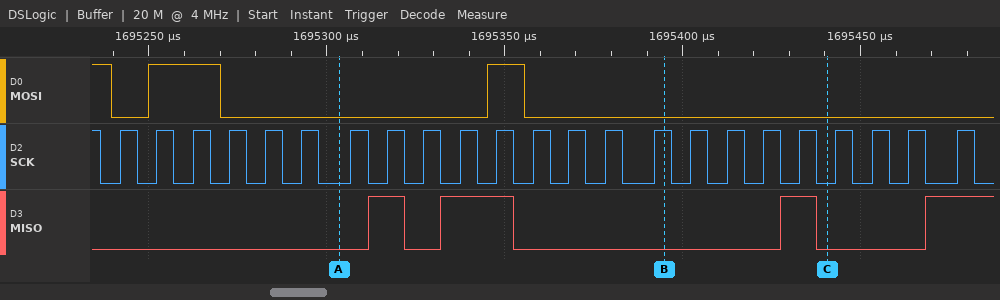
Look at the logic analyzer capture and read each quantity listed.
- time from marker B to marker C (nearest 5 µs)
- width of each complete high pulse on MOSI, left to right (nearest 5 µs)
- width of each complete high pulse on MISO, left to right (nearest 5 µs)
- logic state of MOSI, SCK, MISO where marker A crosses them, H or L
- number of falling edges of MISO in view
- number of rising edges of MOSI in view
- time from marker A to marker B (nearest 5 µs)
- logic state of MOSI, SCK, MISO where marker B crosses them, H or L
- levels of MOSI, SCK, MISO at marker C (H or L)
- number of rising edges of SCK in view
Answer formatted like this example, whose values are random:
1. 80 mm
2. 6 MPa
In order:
1. 45 µs
2. 20 µs, 10 µs
3. 10 µs, 20 µs, 10 µs
4. MOSI=L, SCK=L, MISO=L
5. 3
6. 2
7. 90 µs
8. MOSI=L, SCK=H, MISO=L
9. MOSI=L, SCK=L, MISO=L
10. 23
